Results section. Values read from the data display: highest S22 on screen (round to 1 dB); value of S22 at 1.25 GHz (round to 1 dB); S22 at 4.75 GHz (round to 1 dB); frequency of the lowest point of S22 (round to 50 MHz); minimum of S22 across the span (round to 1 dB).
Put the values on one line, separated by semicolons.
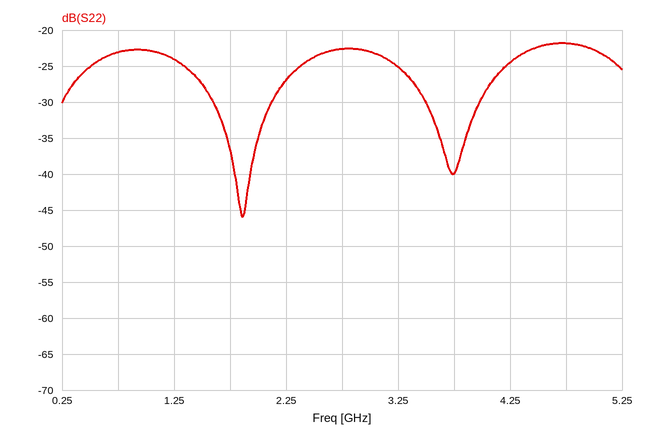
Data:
-22 dB; -24 dB; -22 dB; 1.85 GHz; -46 dB
